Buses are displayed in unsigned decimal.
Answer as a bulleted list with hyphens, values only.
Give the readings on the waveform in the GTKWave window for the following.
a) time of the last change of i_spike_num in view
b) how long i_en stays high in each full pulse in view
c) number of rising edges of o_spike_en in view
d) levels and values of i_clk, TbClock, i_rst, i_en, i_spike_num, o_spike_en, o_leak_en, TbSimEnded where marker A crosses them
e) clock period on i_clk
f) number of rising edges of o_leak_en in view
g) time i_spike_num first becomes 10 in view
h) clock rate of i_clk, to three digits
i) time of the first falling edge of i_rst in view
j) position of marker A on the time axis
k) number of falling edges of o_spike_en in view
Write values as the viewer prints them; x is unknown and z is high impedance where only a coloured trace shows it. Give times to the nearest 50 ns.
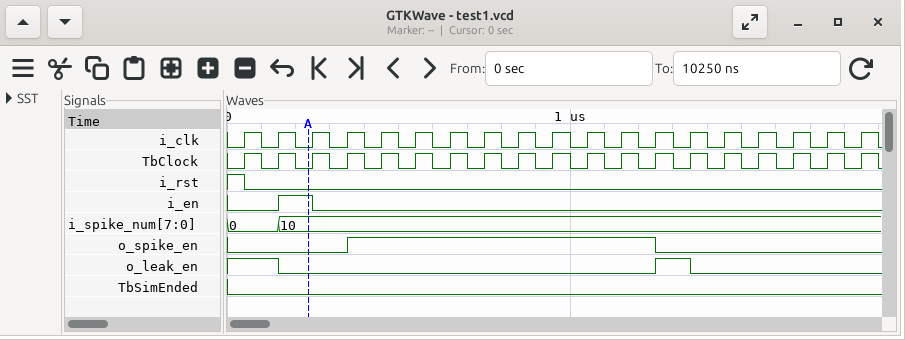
- 150 ns
- 100 ns
- 1
- i_clk=0, TbClock=0, i_rst=0, i_en=1, i_spike_num=10, o_spike_en=0, o_leak_en=0, TbSimEnded=0
- 100 ns
- 1
- 150 ns
- 10.0 MHz
- 50 ns
- 250 ns
- 1
